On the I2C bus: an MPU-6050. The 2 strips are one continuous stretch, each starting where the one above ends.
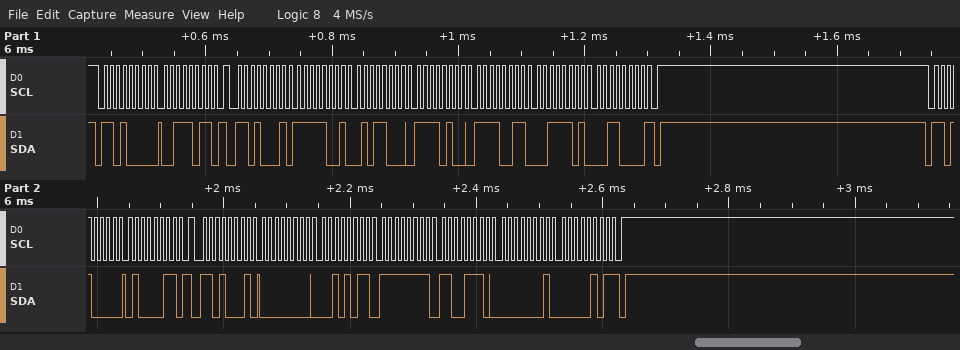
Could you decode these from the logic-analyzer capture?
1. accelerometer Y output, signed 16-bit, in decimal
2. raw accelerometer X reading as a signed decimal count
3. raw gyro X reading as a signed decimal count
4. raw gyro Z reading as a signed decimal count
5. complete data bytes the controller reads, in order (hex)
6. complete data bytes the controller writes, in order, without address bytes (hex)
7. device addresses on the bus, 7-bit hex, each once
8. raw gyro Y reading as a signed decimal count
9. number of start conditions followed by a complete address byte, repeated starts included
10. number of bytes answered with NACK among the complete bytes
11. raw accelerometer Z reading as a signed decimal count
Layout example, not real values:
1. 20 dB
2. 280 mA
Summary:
1. -2829
2. -1704
3. 43
4. 261
5. F9 58 F4 F3 3D 30 00 2B FF CE 01 05
6. 3B 43
7. 0x68
8. -50
9. 4
10. 2
11. 15664
